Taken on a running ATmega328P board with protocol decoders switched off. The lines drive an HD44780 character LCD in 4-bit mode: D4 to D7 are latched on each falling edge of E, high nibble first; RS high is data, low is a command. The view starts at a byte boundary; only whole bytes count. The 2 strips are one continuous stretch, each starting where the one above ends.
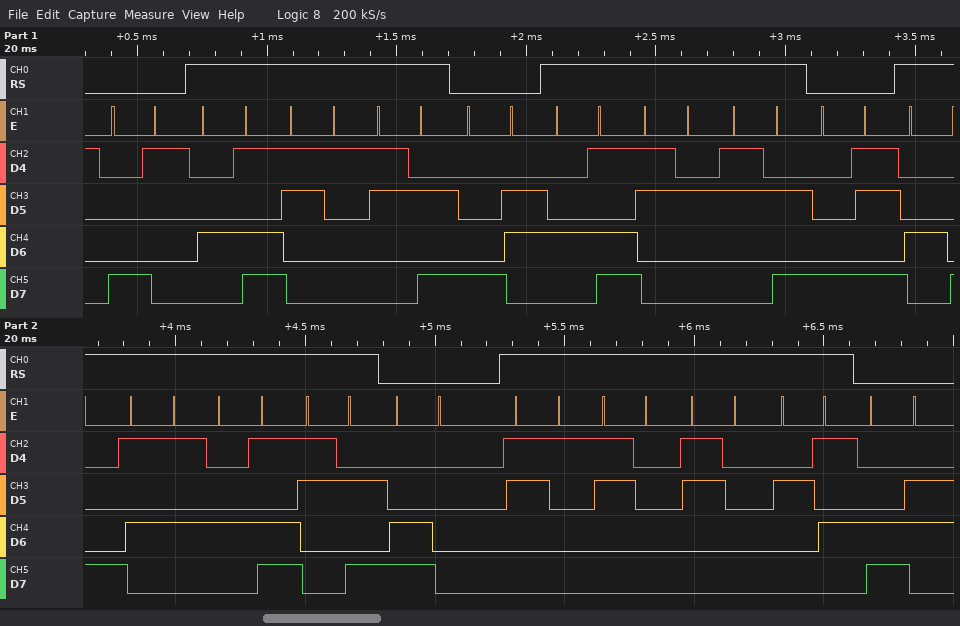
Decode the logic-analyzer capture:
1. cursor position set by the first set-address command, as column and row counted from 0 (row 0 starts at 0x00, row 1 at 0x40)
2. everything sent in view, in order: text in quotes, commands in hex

column 1, row 0
0x81 "M1:" 0x86 "M2:" 0x8B "HUM:" 0xC0 "100%" 0xC6
